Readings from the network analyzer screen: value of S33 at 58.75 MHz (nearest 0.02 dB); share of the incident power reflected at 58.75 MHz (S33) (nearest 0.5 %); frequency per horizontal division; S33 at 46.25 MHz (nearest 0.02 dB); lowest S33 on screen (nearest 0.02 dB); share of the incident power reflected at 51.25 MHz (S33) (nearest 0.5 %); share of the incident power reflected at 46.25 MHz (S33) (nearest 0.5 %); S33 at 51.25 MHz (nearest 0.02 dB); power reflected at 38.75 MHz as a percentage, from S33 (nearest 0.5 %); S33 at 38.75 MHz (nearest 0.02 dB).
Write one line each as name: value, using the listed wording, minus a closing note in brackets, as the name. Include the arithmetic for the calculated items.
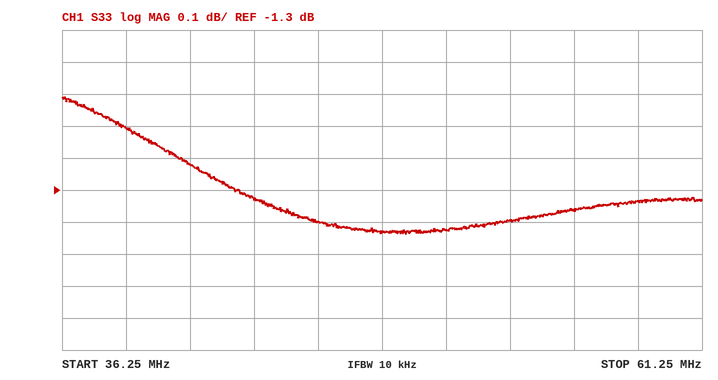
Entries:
value of S33 at 58.75 MHz: -1.34 dB
share of the incident power reflected at 58.75 MHz (S33): 10^(-1.34/10) ≈ 73.5 %
frequency per horizontal division: 2.5 MHz
S33 at 46.25 MHz: -1.40 dB
lowest S33 on screen: -1.44 dB
share of the incident power reflected at 51.25 MHz (S33): 10^(-1.42/10) ≈ 72.1 %, so 72.0 % to the nearest 0.5 %
share of the incident power reflected at 46.25 MHz (S33): 10^(-1.4/10) ≈ 72.4 %, so 72.5 % to the nearest 0.5 %
S33 at 51.25 MHz: -1.42 dB
power reflected at 38.75 MHz as a percentage, from S33: 10^(-1.1/10) ≈ 77.6 %, so 77.5 % to the nearest 0.5 %
S33 at 38.75 MHz: -1.10 dB
